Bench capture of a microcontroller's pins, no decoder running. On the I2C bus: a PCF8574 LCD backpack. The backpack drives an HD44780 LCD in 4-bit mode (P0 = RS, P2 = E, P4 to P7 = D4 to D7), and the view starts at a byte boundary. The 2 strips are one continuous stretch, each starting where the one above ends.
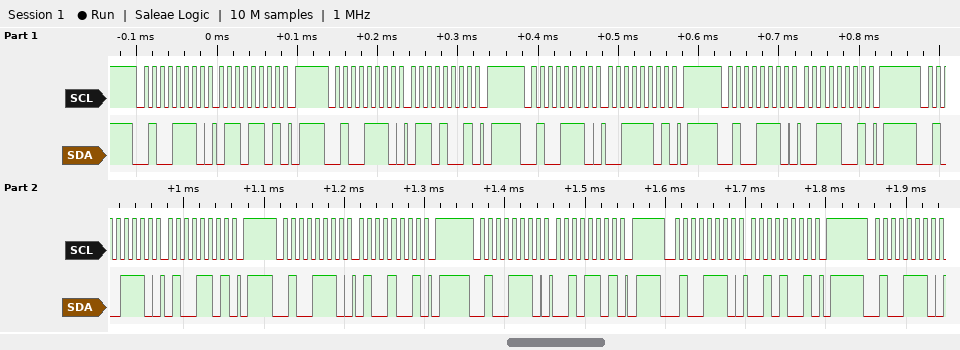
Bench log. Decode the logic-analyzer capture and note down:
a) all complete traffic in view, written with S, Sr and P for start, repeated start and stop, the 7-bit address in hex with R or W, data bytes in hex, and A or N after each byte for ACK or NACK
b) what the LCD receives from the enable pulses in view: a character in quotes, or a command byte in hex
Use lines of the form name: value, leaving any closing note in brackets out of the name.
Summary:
all complete traffic in view, written with S, Sr and P for start, repeated start and stop, the 7-bit address in hex with R or W, data bytes in hex, and A or N after each byte for ACK or NACK: S 27W A 6D A P S 27W A 69 A P S 27W A 3D A P S 27W A 39 A P S 27W A 4D A P S 27W A 49 A P S 27W A 2D A P S 27W A 29 A P S 27W A
what the LCD receives from the enable pulses in view: a character in quotes, or a command byte in hex: 'c' 'B'
